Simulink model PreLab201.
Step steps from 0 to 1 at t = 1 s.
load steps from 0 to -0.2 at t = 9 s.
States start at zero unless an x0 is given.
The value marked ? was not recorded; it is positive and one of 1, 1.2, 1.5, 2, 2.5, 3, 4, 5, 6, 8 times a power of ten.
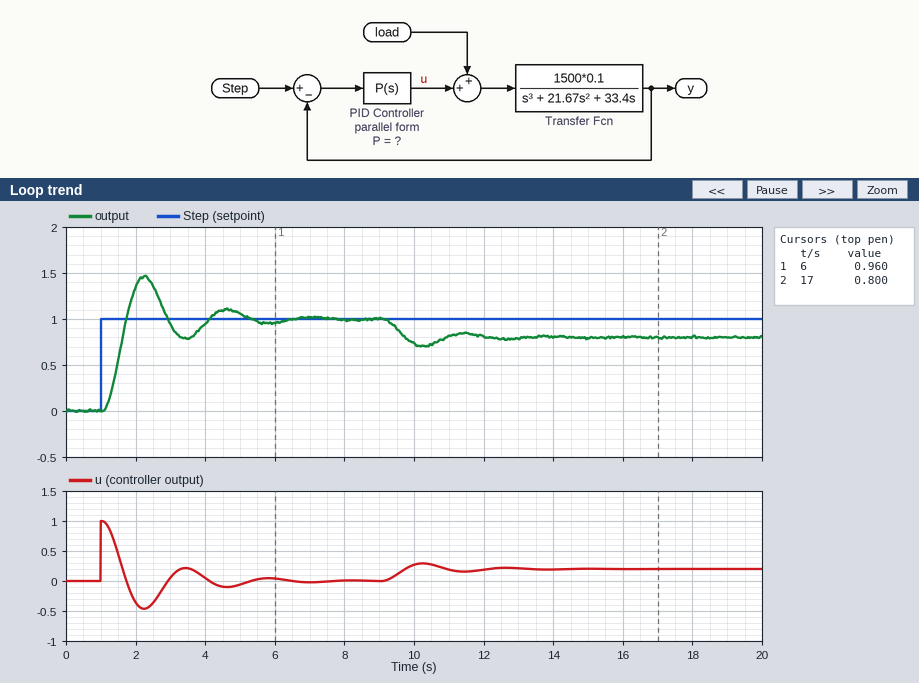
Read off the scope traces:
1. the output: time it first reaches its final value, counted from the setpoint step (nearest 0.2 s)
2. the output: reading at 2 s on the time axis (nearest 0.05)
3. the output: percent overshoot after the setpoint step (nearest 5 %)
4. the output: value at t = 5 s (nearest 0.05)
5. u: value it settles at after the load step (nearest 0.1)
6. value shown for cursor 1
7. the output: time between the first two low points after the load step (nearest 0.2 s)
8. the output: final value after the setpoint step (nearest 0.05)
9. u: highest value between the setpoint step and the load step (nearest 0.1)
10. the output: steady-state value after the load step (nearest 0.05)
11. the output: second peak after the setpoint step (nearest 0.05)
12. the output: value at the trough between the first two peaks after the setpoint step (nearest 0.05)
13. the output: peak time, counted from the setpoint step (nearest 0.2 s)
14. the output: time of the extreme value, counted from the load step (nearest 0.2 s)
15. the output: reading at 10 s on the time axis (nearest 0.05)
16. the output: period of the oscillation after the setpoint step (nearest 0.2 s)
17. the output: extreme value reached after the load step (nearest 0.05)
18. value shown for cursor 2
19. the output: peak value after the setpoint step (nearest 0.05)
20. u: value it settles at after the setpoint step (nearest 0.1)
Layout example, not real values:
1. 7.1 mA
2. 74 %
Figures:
1. 0.8 s
2. 1.35
3. 45 %
4. 1.05
5. 0.2
6. 0.960
7. 2.4 s
8. 1.00
9. 1.0
10. 0.80
11. 1.10
12. 0.80
13. 1.2 s
14. 1.2 s
15. 0.75
16. 2.4 s
17. 0.70
18. 0.800
19. 1.45
20. 0.0
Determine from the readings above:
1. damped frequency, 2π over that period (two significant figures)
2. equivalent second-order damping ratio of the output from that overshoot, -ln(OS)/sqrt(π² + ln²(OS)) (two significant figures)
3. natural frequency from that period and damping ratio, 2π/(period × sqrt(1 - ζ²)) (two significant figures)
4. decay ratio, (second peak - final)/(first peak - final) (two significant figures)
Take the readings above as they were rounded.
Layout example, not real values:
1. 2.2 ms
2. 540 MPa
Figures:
1. 2.6 rad/s
2. 0.25
3. 2.7 rad/s
4. 0.22
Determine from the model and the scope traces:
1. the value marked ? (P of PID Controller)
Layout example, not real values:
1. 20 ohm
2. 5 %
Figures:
1. 1
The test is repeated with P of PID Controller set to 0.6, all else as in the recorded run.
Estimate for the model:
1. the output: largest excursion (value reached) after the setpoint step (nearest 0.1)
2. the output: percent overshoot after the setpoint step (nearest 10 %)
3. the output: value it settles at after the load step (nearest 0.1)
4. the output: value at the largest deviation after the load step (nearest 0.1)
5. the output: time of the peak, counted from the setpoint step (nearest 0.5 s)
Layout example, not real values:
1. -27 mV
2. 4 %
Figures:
1. 1.3
2. 30 %
3. 0.7
4. 0.6
5. 1.5 s
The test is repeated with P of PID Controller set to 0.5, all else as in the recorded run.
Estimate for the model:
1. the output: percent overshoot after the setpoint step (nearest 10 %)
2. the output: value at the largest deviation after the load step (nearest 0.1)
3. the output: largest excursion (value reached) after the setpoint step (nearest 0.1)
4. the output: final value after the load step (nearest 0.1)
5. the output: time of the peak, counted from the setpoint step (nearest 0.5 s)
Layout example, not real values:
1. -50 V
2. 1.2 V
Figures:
1. 30 %
2. 0.5
3. 1.3
4. 0.6
5. 2.0 s
